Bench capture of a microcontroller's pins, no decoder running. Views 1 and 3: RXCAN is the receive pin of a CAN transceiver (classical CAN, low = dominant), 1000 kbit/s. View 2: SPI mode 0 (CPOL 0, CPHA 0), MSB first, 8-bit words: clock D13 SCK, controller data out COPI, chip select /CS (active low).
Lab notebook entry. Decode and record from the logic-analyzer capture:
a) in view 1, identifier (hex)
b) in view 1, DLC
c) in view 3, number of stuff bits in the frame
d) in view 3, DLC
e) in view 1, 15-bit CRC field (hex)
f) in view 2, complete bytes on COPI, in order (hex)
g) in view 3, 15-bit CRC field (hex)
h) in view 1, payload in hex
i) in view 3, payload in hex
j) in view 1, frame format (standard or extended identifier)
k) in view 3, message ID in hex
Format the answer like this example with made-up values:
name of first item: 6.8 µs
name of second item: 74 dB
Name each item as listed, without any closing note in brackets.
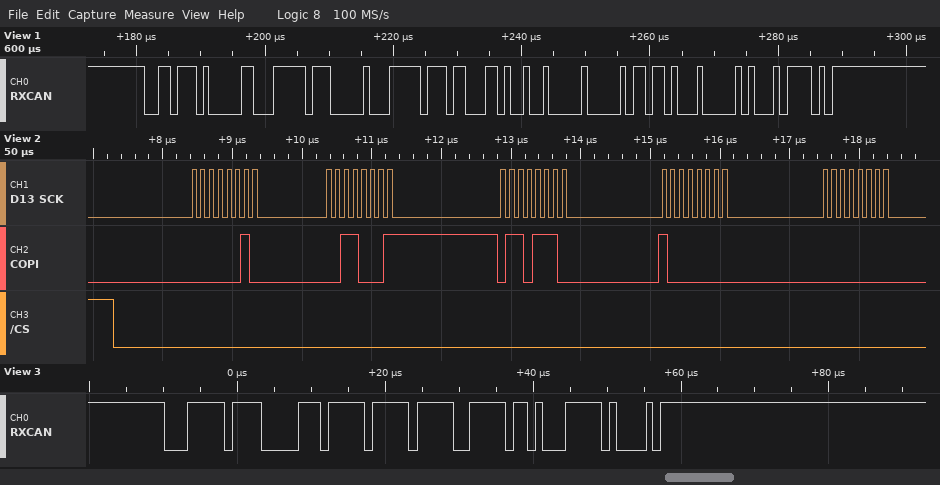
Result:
in view 1, identifier: 0x374
in view 1, DLC: 8
in view 3, number of stuff bits in the frame: 7
in view 3, DLC: 3
in view 1, 15-bit CRC field: 0x045E
in view 2, complete bytes on COPI, in order: 02 31 6E 80 00
in view 3, 15-bit CRC field: 0x23F0
in view 1, payload in hex: FF 00 FF 63 49 00 1B 44
in view 3, payload in hex: 7F FF 7F
in view 1, frame format: standard
in view 3, message ID in hex: 0x1FF
